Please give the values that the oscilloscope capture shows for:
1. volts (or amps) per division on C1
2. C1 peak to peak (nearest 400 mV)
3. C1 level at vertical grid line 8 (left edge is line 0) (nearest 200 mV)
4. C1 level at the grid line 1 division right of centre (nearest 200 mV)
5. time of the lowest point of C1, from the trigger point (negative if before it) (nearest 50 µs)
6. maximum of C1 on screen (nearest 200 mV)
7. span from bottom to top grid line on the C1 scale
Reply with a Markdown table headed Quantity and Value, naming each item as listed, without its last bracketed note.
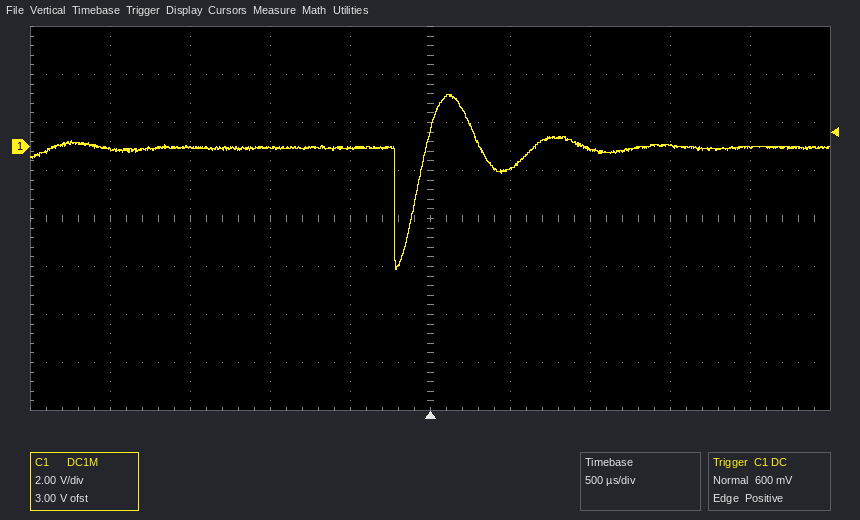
| Quantity | Value |
|---|---|
| volts (or amps) per division on C1 | 2 V |
| C1 peak to peak | 7.2 V |
| C1 level at vertical grid line 8 (left edge is line 0) | 0.0 V |
| C1 level at the grid line 1 division right of centre | -1.0 V |
| time of the lowest point of C1, from the trigger point (negative if before it) | -200 µs |
| maximum of C1 on screen | 2.2 V |
| span from bottom to top grid line on the C1 scale | 16 V |
